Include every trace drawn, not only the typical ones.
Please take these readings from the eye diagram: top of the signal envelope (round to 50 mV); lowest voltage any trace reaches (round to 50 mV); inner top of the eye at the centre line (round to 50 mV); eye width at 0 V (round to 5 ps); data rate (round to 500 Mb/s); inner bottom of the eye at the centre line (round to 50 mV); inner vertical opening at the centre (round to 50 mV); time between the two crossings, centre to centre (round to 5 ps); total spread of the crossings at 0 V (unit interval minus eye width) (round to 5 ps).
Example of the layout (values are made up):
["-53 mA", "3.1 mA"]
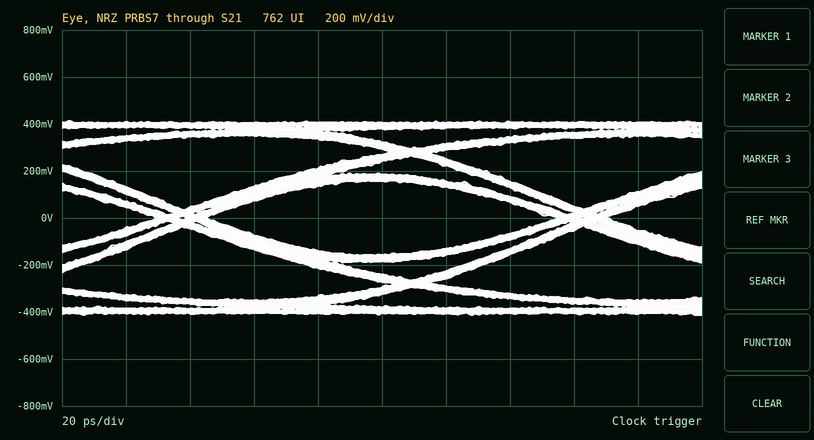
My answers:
["400 mV", "-400 mV", "150 mV", "110 ps", "8.0 Gb/s", "-150 mV", "300 mV", "125 ps", "15 ps"]
